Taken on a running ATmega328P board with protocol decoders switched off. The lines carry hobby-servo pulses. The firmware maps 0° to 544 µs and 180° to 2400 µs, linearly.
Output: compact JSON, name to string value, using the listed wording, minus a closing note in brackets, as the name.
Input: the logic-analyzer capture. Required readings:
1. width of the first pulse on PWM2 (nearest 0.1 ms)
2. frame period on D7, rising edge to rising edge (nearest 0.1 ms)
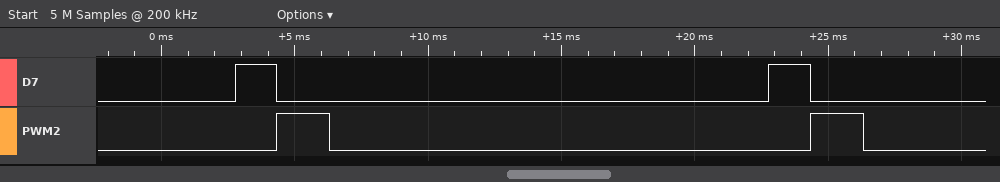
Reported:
{"width of the first pulse on PWM2": "2.0 ms", "frame period on D7, rising edge to rising edge": "20.0 ms"}
